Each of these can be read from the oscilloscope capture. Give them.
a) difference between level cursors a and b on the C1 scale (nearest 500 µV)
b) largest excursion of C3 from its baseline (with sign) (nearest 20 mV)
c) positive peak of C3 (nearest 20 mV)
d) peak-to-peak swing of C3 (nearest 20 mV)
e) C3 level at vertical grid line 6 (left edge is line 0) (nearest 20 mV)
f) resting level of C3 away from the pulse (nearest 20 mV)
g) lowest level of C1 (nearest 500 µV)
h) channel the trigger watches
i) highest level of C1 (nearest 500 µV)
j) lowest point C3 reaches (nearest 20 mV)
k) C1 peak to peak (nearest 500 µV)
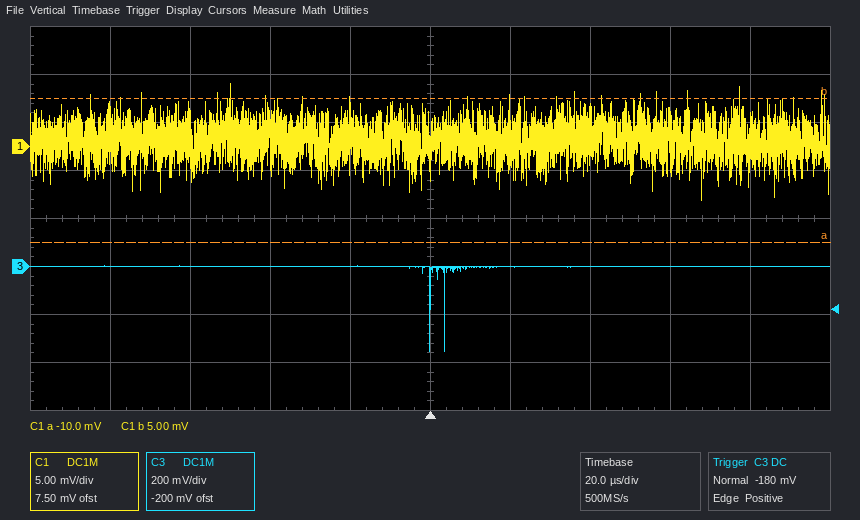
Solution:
15.0 mV
-360 mV
0 mV
360 mV
0 mV
0 mV
-5.5 mV
C3
6.5 mV
-360 mV
12.0 mV
